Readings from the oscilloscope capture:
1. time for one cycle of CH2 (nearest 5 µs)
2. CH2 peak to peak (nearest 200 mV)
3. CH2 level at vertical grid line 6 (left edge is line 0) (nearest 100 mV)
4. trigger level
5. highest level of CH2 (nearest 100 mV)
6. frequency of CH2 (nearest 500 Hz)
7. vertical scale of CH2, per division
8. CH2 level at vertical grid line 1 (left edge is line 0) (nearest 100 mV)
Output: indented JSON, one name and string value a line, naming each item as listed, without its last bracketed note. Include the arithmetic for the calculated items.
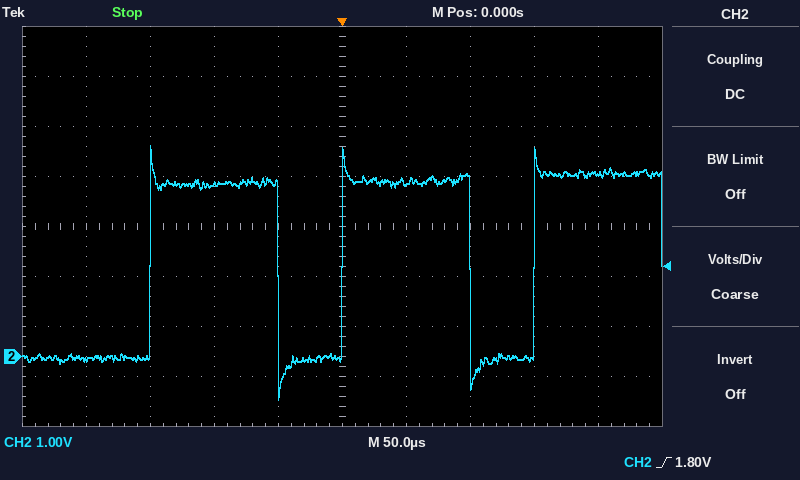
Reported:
{
  "time for one cycle of CH2": "150 µs",
  "CH2 peak to peak": "5.0 V",
  "CH2 level at vertical grid line 6 (left edge is line 0)": "3.5 V",
  "trigger level": "1.80 V",
  "highest level of CH2": "4.2 V",
  "frequency of CH2": "1 / 150 µs ≈ 6.67 kHz, so 6.5 kHz to the nearest 500 Hz",
  "vertical scale of CH2, per division": "1 V",
  "CH2 level at vertical grid line 1 (left edge is line 0)": "-100 mV"
}
